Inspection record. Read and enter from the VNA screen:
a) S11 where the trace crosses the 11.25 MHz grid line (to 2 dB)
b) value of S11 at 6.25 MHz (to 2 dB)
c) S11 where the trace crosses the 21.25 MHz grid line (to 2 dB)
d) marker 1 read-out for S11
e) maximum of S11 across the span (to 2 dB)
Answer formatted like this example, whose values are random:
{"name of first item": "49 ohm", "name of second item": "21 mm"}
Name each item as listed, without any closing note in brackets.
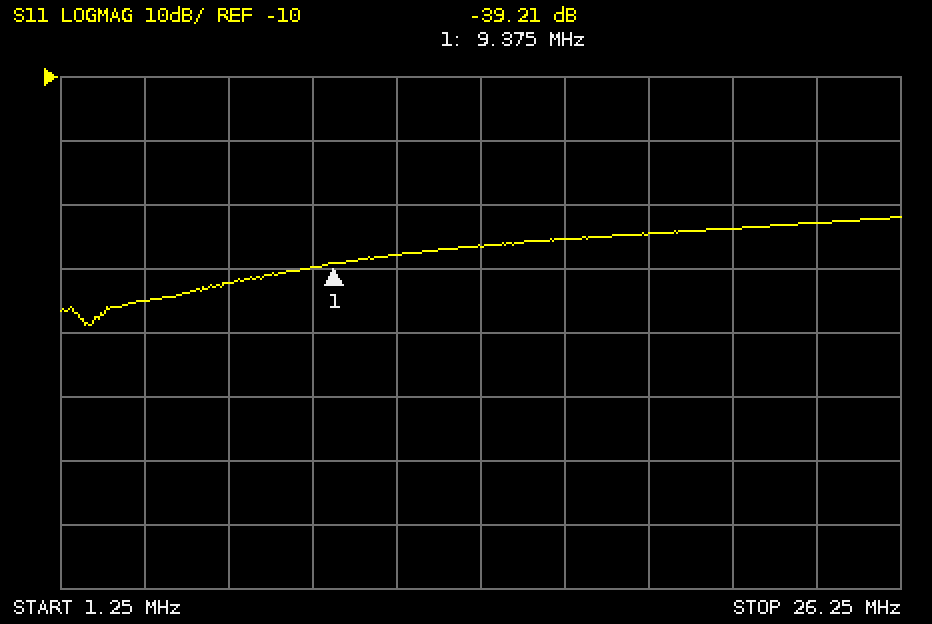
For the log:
{"S11 where the trace crosses the 11.25 MHz grid line": "-38 dB", "value of S11 at 6.25 MHz": "-42 dB", "S11 where the trace crosses the 21.25 MHz grid line": "-34 dB", "marker 1 read-out for S11": "-39.21 dB", "maximum of S11 across the span": "-32 dB"}
